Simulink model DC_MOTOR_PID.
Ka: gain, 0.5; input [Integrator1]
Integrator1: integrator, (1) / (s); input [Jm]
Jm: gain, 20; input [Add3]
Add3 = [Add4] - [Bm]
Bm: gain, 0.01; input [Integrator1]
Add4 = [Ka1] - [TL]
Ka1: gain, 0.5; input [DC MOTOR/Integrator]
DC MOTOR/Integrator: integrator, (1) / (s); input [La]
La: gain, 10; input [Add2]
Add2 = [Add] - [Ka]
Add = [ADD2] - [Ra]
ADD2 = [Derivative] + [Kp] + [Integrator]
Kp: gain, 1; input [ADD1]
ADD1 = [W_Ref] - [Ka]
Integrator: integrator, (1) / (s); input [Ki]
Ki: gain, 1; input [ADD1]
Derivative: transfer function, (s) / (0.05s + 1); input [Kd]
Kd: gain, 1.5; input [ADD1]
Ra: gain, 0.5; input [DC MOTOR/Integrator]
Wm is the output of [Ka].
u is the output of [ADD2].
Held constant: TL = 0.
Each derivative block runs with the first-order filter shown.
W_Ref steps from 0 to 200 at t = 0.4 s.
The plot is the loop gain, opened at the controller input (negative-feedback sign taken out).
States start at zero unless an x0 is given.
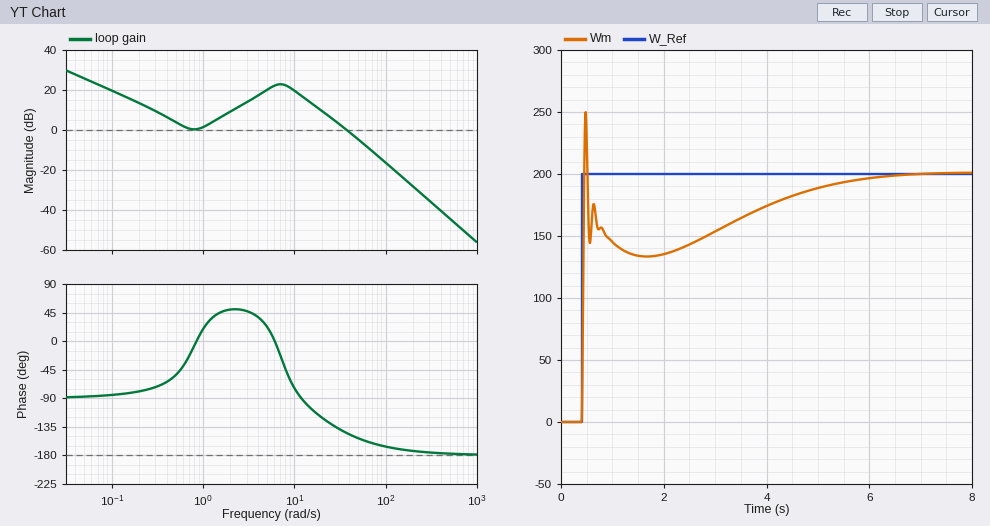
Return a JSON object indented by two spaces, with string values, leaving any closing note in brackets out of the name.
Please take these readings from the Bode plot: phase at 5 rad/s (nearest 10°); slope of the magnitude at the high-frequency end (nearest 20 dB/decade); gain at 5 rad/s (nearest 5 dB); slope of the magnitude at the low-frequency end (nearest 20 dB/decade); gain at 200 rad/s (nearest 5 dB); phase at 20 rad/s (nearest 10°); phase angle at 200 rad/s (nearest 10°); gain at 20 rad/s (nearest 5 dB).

{
  "phase at 5 rad/s": "20°",
  "slope of the magnitude at the high-frequency end": "-40 dB/decade",
  "gain at 5 rad/s": "20 dB",
  "slope of the magnitude at the low-frequency end": "-20 dB/decade",
  "gain at 200 rad/s": "-30 dB",
  "phase at 20 rad/s": "-120°",
  "phase angle at 200 rad/s": "-170°",
  "gain at 20 rad/s": "10 dB"
}
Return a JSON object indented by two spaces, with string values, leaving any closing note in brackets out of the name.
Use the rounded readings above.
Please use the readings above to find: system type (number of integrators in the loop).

{
  "system type": "1"
}
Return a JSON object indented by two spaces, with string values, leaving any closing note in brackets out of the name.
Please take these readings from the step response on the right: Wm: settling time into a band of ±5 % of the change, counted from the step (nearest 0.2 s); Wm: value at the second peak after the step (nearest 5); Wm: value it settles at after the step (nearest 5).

{
  "Wm: settling time into a band of ±5 % of the change, counted from the step": "4.8 s",
  "Wm: value at the second peak after the step": "175",
  "Wm: value it settles at after the step": "200"
}
